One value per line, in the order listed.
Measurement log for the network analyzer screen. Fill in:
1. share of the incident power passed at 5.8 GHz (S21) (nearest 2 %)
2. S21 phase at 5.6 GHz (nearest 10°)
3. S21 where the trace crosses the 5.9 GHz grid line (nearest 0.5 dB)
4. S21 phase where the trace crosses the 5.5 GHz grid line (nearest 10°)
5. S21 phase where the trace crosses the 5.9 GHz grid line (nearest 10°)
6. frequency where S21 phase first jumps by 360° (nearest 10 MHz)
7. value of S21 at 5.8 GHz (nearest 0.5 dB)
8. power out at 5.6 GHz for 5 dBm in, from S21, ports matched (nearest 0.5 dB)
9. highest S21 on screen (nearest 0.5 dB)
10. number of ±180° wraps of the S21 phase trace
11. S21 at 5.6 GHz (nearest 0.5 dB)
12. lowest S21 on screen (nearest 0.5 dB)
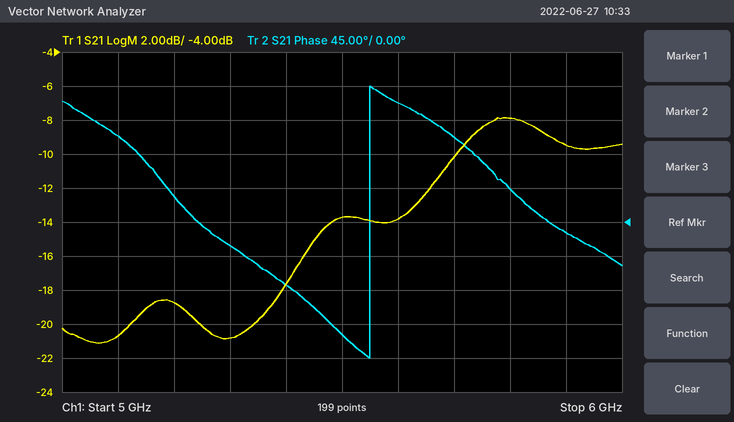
16 %
160°
-9.5 dB
-150°
-10°
5.55 GHz
-8.0 dB
-9.0 dBm
-8.0 dB
1
-14.0 dB
-21.0 dB
